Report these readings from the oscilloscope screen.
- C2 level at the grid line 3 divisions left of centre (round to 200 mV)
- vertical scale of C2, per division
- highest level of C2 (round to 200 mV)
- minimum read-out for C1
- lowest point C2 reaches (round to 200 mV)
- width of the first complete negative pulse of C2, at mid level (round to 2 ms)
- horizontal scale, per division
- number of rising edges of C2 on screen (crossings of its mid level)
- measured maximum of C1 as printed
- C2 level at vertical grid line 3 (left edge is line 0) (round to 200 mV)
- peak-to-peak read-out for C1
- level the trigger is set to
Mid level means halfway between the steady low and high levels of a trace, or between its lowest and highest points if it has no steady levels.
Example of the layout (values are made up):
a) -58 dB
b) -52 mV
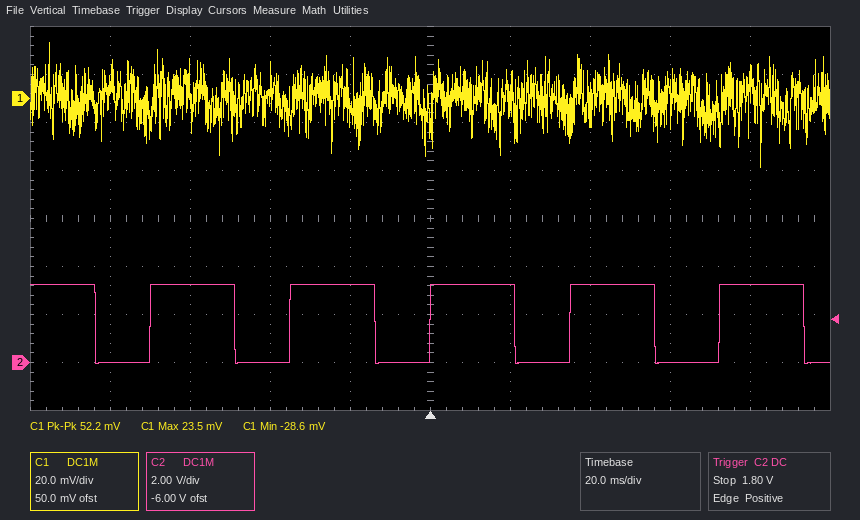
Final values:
a) 3.2 V
b) 2 V
c) 3.2 V
d) -28.6 mV
e) 0.0 V
f) 14 ms
g) 20 ms
h) 5
i) 23.5 mV
j) 0.0 V
k) 52.2 mV
l) 1.80 V
